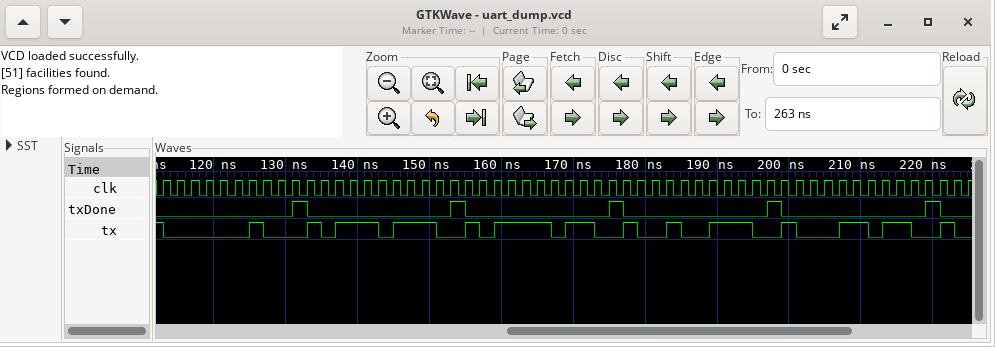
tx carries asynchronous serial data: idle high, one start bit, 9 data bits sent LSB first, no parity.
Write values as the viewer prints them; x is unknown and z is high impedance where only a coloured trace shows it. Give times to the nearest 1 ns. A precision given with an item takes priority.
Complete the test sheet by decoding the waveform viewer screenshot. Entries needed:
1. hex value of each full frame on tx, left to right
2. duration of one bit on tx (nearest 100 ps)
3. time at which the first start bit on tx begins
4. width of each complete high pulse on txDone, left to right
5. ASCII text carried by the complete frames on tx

20, 77, 6F, 72, 6C
2000 ps
113 ns
2 ns, 2 ns, 2 ns, 2 ns, 2 ns
" worl"
